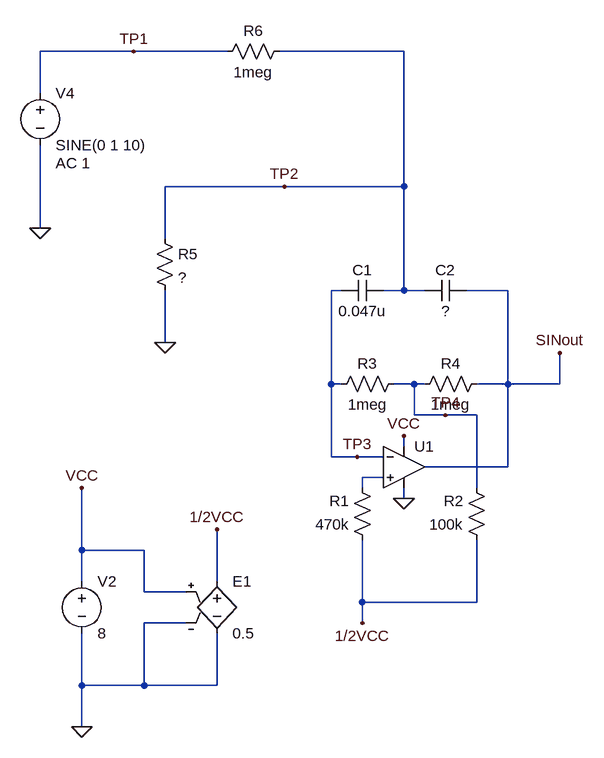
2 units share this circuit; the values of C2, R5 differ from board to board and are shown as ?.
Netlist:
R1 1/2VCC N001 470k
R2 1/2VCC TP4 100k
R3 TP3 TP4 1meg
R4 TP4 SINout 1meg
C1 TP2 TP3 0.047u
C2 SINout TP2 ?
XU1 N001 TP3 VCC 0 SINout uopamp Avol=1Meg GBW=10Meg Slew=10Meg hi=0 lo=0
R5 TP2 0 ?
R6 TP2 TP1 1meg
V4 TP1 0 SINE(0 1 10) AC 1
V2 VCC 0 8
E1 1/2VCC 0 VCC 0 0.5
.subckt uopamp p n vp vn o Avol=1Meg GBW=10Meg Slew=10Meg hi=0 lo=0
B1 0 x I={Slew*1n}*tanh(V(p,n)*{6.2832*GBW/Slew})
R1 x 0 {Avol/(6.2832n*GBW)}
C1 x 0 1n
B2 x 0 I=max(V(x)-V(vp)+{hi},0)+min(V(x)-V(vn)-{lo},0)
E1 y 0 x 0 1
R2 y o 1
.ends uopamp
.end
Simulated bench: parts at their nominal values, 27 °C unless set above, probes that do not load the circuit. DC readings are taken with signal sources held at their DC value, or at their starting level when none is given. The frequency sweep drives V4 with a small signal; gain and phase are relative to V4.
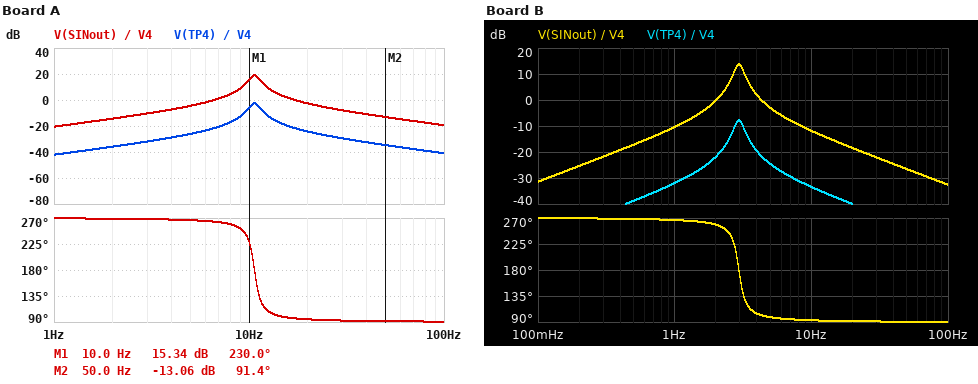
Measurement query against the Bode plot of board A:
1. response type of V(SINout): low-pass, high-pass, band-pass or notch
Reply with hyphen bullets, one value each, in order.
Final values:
- band-pass
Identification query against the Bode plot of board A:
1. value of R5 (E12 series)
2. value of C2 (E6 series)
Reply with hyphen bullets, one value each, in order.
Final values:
- 27 kΩ
- 15 nF
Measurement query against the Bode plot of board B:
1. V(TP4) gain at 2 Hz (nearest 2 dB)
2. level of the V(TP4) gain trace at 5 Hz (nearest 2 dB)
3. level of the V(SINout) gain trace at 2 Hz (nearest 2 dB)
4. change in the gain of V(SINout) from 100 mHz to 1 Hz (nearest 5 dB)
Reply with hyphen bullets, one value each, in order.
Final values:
- -22 dB
- -24 dB
- 0 dB
- 20 dB
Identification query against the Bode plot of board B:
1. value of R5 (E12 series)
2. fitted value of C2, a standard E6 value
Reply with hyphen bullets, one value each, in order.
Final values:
- 82 kΩ
- 68 nF
